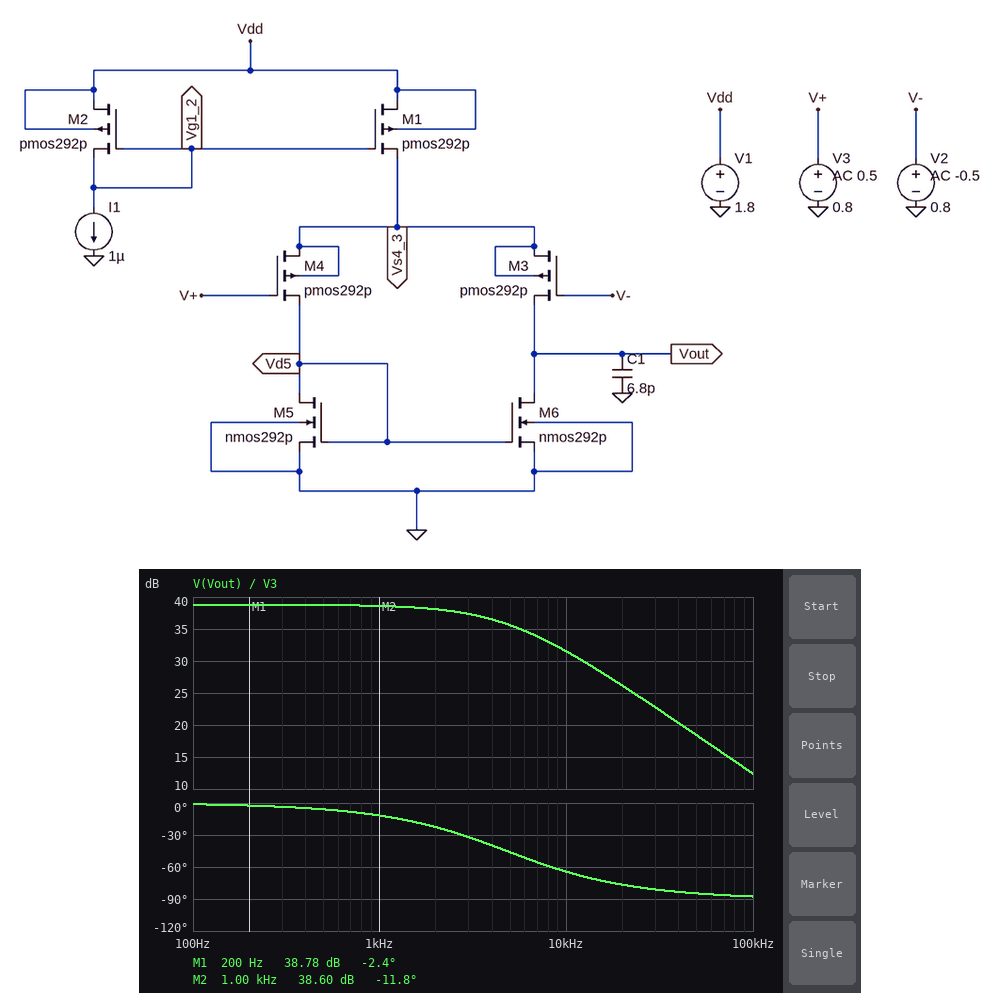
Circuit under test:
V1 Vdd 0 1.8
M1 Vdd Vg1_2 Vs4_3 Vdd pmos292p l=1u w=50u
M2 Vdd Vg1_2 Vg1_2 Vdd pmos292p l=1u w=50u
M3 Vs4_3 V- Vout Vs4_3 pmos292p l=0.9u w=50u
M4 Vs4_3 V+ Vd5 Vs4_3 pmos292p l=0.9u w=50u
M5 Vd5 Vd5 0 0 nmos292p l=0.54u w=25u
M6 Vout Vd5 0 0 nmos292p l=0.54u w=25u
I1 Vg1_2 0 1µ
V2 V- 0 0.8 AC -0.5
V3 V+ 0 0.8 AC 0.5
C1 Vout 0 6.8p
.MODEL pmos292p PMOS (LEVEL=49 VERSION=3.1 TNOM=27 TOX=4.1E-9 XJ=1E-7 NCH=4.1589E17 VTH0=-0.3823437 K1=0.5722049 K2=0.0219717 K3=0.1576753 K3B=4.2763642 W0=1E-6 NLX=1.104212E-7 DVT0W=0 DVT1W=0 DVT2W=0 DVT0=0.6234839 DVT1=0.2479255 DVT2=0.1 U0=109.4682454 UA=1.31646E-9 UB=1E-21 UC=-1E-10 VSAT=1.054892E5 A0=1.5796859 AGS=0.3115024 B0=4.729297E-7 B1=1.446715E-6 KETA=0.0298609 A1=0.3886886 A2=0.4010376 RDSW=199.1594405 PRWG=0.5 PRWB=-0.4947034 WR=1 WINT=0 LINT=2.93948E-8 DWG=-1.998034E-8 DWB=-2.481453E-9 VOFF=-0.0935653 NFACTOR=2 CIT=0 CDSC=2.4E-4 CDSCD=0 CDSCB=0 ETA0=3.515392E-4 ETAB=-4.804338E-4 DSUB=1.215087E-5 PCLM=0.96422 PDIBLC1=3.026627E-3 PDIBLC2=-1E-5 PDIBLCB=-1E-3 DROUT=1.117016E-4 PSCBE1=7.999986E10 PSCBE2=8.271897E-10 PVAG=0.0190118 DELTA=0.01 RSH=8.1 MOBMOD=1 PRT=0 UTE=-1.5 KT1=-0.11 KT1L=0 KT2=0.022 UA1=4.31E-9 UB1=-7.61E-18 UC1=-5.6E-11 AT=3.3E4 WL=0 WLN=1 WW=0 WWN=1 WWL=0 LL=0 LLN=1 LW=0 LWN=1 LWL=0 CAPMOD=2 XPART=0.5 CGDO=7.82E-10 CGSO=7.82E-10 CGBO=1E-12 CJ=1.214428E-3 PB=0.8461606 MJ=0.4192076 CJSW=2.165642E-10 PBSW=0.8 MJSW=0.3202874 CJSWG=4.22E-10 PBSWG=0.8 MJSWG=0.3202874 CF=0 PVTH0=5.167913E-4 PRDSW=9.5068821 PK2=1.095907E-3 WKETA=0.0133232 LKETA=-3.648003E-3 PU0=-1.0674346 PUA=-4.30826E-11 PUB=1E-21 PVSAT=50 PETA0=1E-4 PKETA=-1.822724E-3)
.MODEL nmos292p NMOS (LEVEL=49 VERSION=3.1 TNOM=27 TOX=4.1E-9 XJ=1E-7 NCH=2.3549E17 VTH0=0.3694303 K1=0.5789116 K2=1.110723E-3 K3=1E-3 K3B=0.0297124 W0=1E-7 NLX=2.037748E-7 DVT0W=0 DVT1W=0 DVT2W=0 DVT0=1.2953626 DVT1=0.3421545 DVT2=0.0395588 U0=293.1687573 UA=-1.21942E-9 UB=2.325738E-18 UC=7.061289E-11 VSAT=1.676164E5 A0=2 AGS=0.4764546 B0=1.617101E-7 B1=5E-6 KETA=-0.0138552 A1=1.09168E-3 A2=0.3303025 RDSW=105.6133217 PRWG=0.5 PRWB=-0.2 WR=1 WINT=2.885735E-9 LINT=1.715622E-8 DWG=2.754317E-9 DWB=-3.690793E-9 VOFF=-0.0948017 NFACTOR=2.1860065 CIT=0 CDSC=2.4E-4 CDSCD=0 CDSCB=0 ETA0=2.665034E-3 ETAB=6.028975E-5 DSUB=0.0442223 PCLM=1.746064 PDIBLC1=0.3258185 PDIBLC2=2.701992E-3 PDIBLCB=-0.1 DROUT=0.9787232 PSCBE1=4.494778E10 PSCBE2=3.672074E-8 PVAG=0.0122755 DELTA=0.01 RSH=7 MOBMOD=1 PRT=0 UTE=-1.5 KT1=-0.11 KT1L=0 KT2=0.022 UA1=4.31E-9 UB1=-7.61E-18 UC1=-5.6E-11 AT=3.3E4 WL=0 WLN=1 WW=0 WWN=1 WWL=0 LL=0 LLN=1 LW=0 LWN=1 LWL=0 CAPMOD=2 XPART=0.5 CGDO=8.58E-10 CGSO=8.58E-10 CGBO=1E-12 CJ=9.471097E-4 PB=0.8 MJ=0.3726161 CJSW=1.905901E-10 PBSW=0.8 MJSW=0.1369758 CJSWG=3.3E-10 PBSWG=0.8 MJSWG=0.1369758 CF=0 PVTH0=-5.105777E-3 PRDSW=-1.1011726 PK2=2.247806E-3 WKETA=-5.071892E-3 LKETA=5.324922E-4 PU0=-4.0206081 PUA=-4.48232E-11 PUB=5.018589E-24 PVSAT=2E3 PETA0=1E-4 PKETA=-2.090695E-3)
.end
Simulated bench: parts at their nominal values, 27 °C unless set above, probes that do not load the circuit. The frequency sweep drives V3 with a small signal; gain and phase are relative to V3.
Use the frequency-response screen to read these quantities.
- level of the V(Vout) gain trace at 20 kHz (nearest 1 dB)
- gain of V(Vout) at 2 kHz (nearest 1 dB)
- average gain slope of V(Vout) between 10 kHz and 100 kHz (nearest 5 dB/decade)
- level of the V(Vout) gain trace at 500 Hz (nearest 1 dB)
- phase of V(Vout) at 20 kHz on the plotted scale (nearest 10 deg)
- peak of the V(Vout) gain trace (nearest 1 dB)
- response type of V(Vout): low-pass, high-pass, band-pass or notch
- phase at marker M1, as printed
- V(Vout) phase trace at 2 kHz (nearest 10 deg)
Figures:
26 dB
38 dB
-20 dB/decade
39 dB
-80 deg
39 dB
low-pass
-2.4 deg
-20 deg
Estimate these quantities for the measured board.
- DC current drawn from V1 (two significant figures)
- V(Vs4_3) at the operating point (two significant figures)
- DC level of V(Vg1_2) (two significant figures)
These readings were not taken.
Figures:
2.0 µA
1.1 V
1.4 V
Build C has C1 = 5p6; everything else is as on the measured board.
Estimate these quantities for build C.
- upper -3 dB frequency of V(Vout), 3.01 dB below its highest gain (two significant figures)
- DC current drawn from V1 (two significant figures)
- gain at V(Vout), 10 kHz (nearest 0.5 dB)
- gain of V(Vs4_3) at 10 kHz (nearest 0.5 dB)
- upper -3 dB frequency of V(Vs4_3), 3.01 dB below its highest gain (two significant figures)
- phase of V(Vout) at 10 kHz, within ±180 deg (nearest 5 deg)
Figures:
5.8 kHz
2.0 µA
33.0 dB
-9.5 dB
8.0 kHz
-60 deg
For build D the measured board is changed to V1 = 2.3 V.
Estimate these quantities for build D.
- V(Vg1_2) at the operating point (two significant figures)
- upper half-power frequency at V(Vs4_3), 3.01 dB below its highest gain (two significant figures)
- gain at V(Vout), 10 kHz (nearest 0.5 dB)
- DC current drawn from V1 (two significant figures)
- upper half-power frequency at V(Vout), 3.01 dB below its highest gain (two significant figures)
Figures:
1.9 V
7.0 kHz
32.0 dB
2.1 µA
5.1 kHz
